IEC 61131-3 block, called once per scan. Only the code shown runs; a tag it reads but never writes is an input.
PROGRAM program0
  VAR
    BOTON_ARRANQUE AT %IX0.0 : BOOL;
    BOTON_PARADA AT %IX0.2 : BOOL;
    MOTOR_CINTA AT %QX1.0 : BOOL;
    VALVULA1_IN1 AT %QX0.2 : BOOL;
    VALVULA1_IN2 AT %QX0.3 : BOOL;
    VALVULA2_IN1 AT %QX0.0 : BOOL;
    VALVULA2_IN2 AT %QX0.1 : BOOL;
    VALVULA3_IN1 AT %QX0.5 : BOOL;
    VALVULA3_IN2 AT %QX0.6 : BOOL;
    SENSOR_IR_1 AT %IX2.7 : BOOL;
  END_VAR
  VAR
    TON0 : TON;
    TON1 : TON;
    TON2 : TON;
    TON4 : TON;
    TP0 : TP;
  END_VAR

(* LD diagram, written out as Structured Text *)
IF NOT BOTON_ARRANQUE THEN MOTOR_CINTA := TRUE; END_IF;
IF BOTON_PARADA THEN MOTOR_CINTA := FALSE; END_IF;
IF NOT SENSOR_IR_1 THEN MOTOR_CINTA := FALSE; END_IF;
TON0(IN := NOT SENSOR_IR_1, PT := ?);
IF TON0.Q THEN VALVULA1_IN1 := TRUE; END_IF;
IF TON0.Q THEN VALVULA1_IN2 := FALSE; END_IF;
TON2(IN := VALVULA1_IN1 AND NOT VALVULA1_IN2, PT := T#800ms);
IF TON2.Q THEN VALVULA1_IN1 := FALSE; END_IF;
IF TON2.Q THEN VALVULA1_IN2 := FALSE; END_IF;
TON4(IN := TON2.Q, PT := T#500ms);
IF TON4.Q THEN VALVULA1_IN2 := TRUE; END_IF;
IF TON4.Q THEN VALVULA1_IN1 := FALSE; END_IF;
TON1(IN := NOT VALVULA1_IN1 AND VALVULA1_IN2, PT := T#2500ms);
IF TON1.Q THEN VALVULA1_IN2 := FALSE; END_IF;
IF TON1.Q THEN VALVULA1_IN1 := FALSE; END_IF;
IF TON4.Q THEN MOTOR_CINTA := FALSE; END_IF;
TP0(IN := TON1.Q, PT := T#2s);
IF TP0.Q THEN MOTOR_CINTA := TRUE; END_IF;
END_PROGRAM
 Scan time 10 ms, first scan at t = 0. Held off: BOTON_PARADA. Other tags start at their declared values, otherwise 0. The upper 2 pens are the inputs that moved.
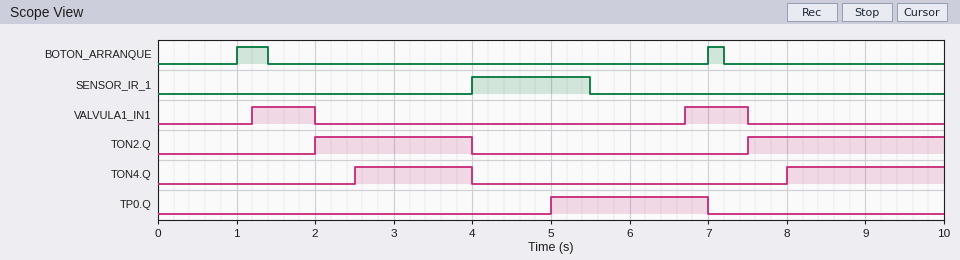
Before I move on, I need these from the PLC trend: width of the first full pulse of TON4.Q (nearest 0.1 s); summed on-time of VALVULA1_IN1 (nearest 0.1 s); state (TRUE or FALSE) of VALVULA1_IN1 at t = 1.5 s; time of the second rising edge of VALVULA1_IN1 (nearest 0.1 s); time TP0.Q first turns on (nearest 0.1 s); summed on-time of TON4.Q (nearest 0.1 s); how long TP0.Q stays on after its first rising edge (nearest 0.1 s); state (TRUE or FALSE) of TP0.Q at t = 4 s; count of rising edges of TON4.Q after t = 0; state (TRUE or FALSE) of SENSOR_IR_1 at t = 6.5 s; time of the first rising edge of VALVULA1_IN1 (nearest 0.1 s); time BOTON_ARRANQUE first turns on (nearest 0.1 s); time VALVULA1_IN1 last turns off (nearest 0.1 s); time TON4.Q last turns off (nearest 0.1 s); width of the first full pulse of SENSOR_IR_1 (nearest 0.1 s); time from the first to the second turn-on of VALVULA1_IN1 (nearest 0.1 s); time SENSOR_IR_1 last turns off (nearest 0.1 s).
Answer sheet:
1.5 s
1.6 s
TRUE
6.7 s
5.0 s
3.5 s
2.0 s
FALSE
2
FALSE
1.2 s
1.0 s
7.5 s
4.0 s
1.5 s
5.5 s
5.5 s
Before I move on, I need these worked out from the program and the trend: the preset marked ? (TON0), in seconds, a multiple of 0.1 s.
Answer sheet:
1.2 s
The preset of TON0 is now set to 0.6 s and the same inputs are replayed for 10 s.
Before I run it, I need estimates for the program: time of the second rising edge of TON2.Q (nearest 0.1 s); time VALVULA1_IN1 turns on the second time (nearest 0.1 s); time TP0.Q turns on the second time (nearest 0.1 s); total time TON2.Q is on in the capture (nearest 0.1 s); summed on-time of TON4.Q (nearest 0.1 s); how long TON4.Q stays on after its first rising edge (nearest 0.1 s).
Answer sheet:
6.9 s
6.1 s
9.9 s
5.7 s
4.7 s
2.1 s
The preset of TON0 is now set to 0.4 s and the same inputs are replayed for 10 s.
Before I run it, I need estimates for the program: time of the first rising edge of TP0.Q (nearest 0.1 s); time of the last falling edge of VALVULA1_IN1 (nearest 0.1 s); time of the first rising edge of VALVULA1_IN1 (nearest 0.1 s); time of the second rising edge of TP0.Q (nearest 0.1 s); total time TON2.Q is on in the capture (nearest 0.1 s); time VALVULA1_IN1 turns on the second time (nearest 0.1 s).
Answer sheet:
4.2 s
6.7 s
0.4 s
9.7 s
6.1 s
5.9 s
